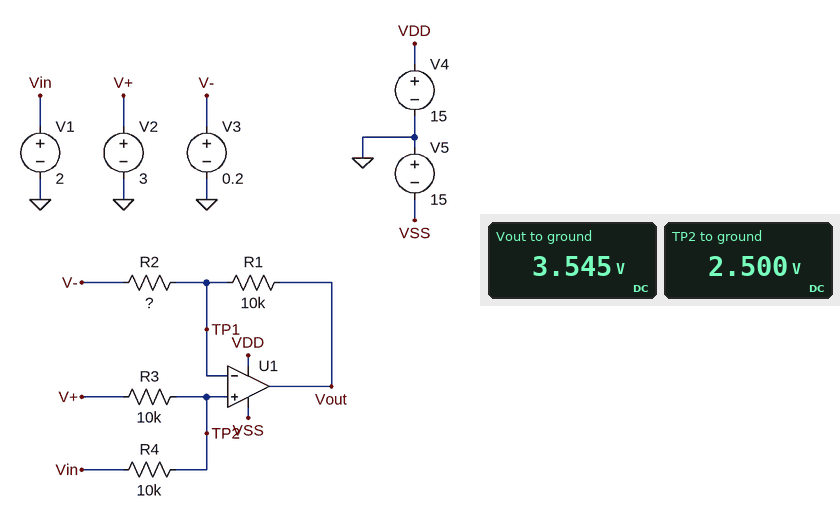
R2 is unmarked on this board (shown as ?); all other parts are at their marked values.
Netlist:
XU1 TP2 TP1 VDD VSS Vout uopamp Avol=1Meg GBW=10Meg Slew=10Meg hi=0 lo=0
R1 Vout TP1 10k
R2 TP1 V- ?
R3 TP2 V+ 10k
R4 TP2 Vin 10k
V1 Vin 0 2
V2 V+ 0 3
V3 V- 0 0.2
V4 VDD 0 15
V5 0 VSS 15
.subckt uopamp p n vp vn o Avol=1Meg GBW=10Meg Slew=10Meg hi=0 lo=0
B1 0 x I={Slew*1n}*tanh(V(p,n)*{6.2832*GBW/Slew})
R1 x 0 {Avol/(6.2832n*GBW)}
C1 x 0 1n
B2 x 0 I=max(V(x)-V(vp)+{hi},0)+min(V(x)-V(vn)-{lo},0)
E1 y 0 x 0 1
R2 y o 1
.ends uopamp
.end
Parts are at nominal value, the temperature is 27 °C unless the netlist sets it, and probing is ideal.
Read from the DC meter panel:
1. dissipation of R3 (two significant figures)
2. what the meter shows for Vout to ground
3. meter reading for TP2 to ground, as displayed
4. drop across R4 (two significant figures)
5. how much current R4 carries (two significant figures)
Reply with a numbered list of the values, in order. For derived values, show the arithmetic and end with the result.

1. (3 V - 2.5 V)^2 / 10 kΩ = 25 µW
2. 3.545 V
3. 2.500 V
4. 2.5 V - 2 V = 500 mV
5. (2.5 V - 2 V) / 10 kΩ = 50 µA
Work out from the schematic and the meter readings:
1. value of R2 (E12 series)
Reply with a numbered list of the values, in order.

1. 22 kΩ
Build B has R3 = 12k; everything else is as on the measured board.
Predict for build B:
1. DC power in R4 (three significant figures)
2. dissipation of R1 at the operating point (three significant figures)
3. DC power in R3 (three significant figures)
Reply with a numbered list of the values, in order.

1. 20.7 µW
2. 105 µW
3. 24.8 µW
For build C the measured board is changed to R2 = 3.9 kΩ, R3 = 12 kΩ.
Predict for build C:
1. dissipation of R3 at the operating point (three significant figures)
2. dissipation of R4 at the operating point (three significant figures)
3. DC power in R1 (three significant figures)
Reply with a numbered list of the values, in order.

1. 24.8 µW
2. 20.7 µW
3. 3.34 mW
